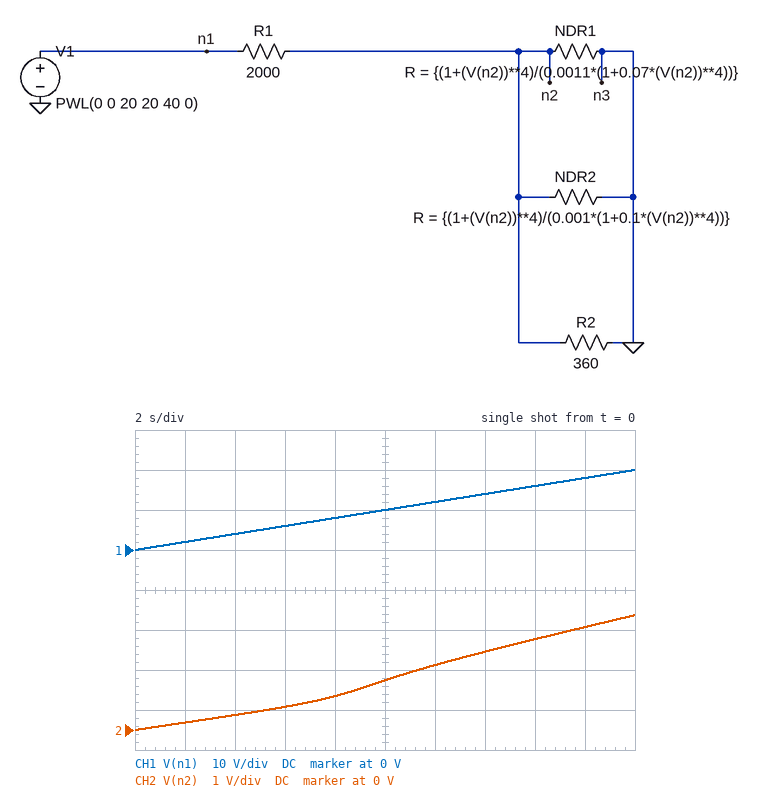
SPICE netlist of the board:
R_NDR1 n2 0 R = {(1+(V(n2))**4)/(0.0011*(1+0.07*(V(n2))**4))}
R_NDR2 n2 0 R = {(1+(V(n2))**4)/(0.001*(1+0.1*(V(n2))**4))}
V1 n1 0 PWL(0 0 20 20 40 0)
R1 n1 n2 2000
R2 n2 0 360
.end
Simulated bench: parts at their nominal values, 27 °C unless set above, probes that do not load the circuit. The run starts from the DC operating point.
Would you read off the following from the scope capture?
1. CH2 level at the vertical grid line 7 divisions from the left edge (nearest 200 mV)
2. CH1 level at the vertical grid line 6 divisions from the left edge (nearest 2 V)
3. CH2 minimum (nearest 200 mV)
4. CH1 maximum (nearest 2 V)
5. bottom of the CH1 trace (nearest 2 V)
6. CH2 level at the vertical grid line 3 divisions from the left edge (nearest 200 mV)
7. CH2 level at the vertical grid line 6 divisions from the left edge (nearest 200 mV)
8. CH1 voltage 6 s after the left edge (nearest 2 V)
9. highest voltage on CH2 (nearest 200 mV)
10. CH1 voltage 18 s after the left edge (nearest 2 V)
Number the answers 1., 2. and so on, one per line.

1. 2.0 V
2. 12 V
3. 0 V
4. 20 V
5. 0 V
6. 600 mV
7. 1.6 V
8. 6 V
9. 2.8 V
10. 18 V
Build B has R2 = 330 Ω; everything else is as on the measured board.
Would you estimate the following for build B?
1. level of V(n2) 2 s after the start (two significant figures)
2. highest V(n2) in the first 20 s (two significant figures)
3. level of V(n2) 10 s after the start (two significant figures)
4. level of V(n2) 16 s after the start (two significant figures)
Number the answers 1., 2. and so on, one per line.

1. 180 mV
2. 2.7 V
3. 1.1 V
4. 2.1 V
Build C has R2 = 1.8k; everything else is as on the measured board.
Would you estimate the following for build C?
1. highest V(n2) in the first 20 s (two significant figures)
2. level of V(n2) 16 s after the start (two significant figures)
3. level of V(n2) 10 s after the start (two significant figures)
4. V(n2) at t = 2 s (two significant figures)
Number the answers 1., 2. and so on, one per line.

1. 8.1 V
2. 6.5 V
3. 4.0 V
4. 320 mV
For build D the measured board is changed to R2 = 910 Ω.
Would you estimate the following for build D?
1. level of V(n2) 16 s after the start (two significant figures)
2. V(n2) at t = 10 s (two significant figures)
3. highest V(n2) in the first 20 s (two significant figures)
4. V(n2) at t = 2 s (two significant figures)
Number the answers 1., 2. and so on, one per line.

1. 4.5 V
2. 2.8 V
3. 5.6 V
4. 270 mV
